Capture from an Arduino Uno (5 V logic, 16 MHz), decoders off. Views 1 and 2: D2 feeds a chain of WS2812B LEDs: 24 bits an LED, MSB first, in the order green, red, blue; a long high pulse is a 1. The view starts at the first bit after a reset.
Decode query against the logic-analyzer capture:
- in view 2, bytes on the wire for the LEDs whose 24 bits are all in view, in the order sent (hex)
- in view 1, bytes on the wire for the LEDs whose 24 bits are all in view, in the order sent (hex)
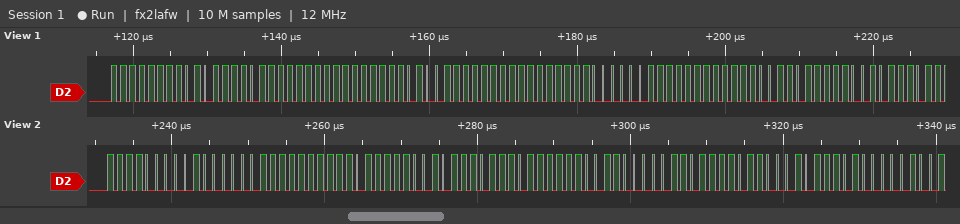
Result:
F0 40 FF DF 2E EF CC 1B D8
FF 5E FF FF 4F FF F0 3F FC
